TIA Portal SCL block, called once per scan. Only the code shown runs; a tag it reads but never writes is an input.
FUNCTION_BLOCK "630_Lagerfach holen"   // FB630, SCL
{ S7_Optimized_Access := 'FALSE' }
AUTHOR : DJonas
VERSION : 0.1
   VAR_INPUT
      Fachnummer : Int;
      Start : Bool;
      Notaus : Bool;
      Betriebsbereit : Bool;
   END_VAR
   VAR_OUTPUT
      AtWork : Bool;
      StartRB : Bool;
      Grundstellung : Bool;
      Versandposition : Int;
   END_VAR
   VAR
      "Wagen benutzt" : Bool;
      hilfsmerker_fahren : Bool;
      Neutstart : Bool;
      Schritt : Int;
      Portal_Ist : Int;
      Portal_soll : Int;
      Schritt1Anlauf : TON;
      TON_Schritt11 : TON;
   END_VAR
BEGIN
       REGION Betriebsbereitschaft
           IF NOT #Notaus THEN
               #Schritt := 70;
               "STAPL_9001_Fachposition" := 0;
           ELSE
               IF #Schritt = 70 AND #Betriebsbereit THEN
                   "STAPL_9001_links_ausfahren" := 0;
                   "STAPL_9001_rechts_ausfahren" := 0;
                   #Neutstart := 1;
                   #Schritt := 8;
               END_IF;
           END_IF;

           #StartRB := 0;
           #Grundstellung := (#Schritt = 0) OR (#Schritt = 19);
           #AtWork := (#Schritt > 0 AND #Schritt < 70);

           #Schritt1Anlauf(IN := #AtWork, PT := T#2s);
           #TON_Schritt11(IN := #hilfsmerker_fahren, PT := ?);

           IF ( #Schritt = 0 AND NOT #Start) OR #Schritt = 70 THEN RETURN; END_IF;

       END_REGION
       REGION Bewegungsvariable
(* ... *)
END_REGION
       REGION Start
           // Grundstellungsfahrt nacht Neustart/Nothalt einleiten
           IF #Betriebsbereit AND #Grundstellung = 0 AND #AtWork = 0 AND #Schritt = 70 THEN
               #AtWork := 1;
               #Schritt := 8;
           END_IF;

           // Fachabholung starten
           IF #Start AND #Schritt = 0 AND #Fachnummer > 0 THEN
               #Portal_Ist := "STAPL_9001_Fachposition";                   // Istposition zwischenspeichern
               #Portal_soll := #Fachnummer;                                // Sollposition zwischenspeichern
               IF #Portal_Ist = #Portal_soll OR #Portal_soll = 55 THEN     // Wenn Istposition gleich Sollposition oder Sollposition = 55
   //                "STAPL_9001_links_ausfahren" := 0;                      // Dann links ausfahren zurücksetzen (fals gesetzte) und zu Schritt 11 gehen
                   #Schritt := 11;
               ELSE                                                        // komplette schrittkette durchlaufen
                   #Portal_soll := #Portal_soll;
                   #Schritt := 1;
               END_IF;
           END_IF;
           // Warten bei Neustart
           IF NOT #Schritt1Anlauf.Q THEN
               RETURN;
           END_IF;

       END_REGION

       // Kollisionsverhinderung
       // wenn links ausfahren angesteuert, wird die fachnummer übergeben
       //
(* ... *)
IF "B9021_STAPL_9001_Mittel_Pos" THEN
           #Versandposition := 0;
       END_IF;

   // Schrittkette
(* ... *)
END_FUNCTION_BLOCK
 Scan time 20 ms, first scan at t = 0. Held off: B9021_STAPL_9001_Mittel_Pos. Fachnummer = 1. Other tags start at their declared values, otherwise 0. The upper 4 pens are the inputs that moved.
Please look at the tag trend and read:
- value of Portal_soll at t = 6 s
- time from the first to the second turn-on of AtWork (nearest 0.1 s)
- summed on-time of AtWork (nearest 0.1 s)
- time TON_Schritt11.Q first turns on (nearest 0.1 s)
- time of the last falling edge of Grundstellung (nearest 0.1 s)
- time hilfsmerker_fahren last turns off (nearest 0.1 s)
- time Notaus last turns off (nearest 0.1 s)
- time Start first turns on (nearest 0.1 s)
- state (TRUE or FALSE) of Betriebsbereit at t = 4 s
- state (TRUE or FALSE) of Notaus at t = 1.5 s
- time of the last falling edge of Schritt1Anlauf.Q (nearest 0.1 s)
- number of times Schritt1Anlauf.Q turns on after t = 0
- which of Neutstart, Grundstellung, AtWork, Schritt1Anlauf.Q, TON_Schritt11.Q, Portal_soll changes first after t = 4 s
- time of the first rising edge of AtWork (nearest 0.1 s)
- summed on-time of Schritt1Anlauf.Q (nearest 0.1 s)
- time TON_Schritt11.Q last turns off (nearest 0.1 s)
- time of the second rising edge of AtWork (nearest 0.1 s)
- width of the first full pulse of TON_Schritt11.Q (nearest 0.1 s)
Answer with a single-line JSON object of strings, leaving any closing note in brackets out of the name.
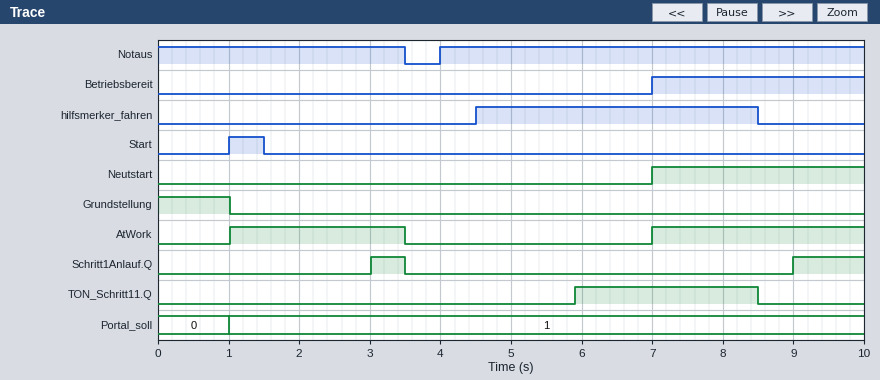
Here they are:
{"value of Portal_soll at t = 6 s": "1", "time from the first to the second turn-on of AtWork": "6.0 s", "summed on-time of AtWork": "5.5 s", "time TON_Schritt11.Q first turns on": "5.9 s", "time of the last falling edge of Grundstellung": "1.0 s", "time hilfsmerker_fahren last turns off": "8.5 s", "time Notaus last turns off": "3.5 s", "time Start first turns on": "1.0 s", "state (TRUE or FALSE) of Betriebsbereit at t = 4 s": "FALSE", "state (TRUE or FALSE) of Notaus at t = 1.5 s": "TRUE", "time of the last falling edge of Schritt1Anlauf.Q": "3.5 s", "number of times Schritt1Anlauf.Q turns on after t = 0": "2", "which of Neutstart, Grundstellung, AtWork, Schritt1Anlauf.Q, TON_Schritt11.Q, Portal_soll changes first after t = 4 s": "TON_Schritt11.Q", "time of the first rising edge of AtWork": "1.0 s", "summed on-time of Schritt1Anlauf.Q": "1.5 s", "time TON_Schritt11.Q last turns off": "8.5 s", "time of the second rising edge of AtWork": "7.0 s", "width of the first full pulse of TON_Schritt11.Q": "2.6 s"}
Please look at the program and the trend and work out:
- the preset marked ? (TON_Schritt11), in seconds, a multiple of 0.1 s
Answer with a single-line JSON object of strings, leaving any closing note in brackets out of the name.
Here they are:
{"the preset marked ? (TON_Schritt11), in seconds, a multiple of 0.1 s": "1.4 s"}
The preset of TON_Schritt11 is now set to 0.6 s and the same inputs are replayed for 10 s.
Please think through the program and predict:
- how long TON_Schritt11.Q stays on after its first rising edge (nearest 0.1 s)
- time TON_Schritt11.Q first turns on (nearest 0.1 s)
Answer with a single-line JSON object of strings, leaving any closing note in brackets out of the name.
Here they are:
{"how long TON_Schritt11.Q stays on after its first rising edge": "3.4 s", "time TON_Schritt11.Q first turns on": "5.1 s"}
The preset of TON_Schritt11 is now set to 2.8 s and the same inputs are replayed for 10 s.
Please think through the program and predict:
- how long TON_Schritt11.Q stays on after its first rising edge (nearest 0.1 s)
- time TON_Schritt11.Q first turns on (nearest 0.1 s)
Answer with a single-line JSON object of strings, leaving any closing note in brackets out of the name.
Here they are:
{"how long TON_Schritt11.Q stays on after its first rising edge": "1.2 s", "time TON_Schritt11.Q first turns on": "7.3 s"}
